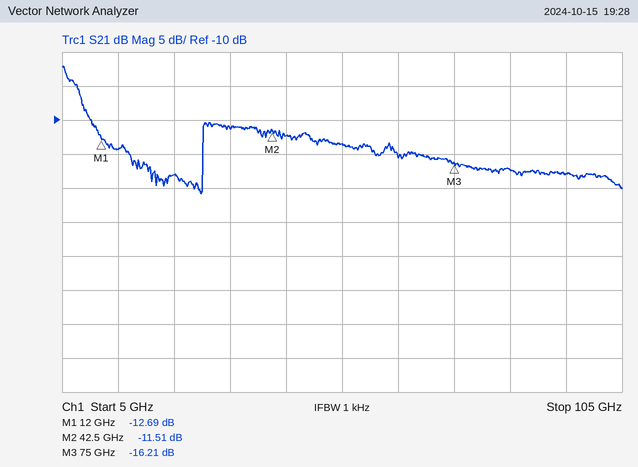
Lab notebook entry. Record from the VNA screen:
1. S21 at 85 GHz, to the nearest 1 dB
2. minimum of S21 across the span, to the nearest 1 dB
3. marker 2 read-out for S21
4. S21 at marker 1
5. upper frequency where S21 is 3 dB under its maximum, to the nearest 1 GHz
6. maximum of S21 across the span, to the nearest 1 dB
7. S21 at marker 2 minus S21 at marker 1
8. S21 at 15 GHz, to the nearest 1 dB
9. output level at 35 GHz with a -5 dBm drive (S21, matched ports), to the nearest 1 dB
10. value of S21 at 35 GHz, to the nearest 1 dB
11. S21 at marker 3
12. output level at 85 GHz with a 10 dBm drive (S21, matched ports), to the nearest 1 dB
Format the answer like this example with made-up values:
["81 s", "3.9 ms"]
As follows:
["-17 dB", "-21 dB", "-11.51 dB", "-12.69 dB", "8 GHz", "-2 dB", "1.18 dB", "-14 dB", "-16 dBm", "-11 dB", "-16.21 dB", "-7 dBm"]
